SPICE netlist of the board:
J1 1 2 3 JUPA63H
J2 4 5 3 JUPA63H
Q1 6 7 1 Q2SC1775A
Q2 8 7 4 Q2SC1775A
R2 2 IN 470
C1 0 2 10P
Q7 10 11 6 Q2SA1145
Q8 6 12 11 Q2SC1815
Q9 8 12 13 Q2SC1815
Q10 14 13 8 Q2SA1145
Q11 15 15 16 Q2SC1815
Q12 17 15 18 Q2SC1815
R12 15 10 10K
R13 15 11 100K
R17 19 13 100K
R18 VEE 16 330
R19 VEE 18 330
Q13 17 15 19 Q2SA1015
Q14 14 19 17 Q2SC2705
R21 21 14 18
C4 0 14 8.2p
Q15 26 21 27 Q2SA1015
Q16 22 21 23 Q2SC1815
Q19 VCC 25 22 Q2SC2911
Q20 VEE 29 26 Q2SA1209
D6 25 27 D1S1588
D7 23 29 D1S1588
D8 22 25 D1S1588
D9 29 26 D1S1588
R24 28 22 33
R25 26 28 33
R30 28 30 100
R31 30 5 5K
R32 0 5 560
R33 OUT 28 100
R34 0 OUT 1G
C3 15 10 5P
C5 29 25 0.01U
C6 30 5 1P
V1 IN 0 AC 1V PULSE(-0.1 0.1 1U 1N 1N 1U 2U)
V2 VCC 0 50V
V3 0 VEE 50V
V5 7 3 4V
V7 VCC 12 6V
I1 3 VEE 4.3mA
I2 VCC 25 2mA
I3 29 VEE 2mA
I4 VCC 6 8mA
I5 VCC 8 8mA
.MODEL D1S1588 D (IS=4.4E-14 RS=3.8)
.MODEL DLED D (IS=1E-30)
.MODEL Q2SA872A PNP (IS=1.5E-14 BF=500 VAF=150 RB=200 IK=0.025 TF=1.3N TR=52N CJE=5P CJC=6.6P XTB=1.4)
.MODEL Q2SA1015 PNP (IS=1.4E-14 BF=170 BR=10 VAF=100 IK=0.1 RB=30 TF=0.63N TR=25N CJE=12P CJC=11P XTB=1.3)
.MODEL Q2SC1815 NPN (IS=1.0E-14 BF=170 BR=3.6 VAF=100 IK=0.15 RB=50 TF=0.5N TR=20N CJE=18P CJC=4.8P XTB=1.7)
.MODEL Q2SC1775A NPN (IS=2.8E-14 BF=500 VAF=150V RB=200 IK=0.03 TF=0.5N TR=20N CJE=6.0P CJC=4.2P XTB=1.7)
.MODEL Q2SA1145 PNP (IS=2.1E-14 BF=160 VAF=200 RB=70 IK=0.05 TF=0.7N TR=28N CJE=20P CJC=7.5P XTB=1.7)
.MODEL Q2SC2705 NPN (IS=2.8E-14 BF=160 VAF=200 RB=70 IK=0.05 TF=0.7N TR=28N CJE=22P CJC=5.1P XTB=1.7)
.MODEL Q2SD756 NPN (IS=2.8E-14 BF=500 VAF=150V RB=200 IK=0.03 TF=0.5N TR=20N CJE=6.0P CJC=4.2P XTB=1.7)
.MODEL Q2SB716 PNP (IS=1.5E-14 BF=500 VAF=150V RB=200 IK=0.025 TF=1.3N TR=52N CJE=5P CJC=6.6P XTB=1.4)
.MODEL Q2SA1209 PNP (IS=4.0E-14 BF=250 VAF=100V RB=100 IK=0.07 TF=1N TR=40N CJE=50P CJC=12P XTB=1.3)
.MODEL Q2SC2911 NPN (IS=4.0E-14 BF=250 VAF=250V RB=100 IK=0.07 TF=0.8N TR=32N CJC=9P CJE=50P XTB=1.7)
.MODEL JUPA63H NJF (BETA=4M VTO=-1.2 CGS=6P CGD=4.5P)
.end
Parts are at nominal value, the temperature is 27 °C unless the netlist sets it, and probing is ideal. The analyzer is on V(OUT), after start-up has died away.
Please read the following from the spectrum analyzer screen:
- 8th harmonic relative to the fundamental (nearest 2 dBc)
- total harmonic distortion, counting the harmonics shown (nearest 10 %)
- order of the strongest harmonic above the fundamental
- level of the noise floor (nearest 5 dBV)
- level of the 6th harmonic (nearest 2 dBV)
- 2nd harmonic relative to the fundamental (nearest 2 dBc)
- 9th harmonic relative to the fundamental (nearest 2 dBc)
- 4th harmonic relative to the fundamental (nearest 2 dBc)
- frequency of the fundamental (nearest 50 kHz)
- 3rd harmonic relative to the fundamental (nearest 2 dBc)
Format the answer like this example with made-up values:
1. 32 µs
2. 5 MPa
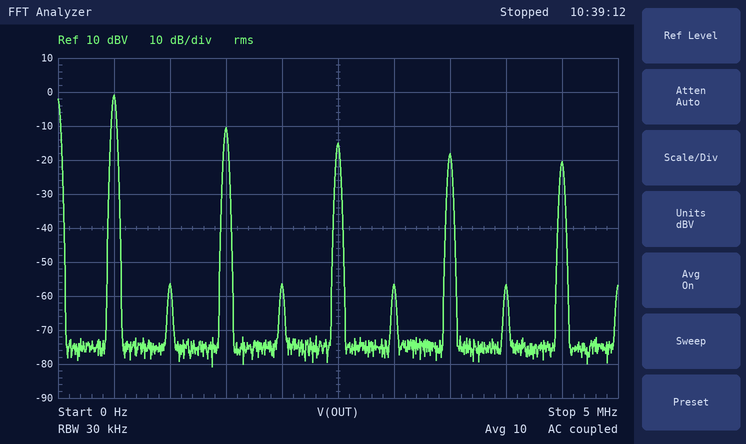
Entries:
1. -56 dBc
2. 40 %
3. 3
4. -75 dBV
5. -56 dBV
6. -56 dBc
7. -20 dBc
8. -56 dBc
9. 500 kHz
10. -10 dBc
